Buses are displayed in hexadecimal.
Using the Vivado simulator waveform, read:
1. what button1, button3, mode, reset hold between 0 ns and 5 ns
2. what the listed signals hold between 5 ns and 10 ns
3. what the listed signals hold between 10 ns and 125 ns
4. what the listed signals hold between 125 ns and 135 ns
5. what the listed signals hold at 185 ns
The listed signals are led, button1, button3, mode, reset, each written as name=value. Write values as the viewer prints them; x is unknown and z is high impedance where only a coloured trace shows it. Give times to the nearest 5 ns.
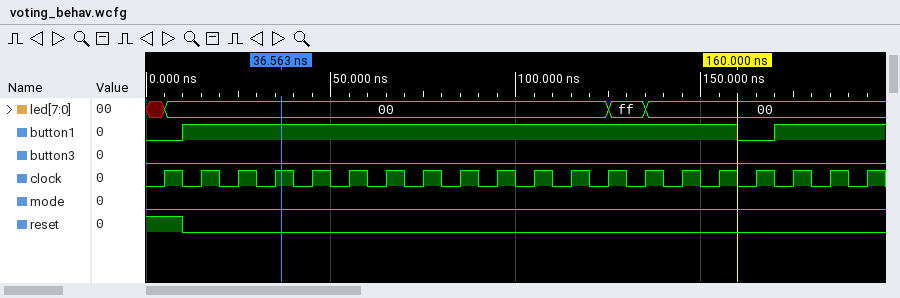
button1=0, button3=0, mode=0, reset=1
led=00, button1=0, button3=0, mode=0, reset=1
led=00, button1=1, button3=0, mode=0, reset=0
led=ff, button1=1, button3=0, mode=0, reset=0
led=00, button1=1, button3=0, mode=0, reset=0
